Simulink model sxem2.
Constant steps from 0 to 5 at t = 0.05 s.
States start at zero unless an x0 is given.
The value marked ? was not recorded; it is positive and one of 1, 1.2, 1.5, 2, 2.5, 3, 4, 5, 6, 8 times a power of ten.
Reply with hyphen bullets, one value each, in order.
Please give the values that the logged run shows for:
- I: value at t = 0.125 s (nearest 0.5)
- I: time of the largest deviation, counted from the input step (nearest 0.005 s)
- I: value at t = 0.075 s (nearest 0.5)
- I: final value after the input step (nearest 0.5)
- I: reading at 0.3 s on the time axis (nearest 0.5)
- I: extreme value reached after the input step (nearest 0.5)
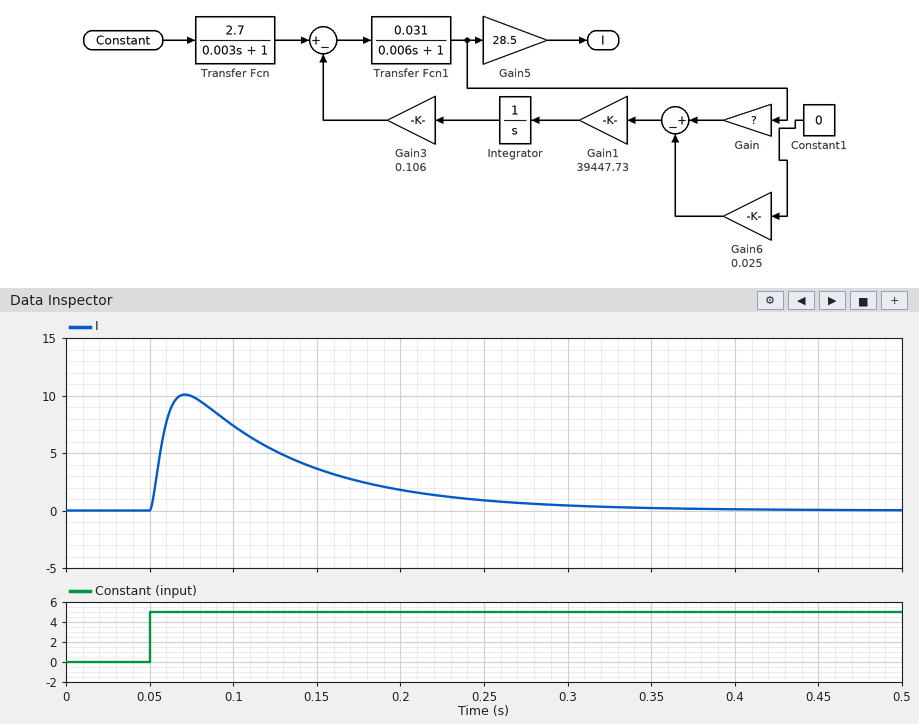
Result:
- 5.0
- 0.020 s
- 10.0
- 0.0
- 0.5
- 10.0
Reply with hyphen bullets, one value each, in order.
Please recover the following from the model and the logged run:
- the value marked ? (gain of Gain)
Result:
- 0.1
